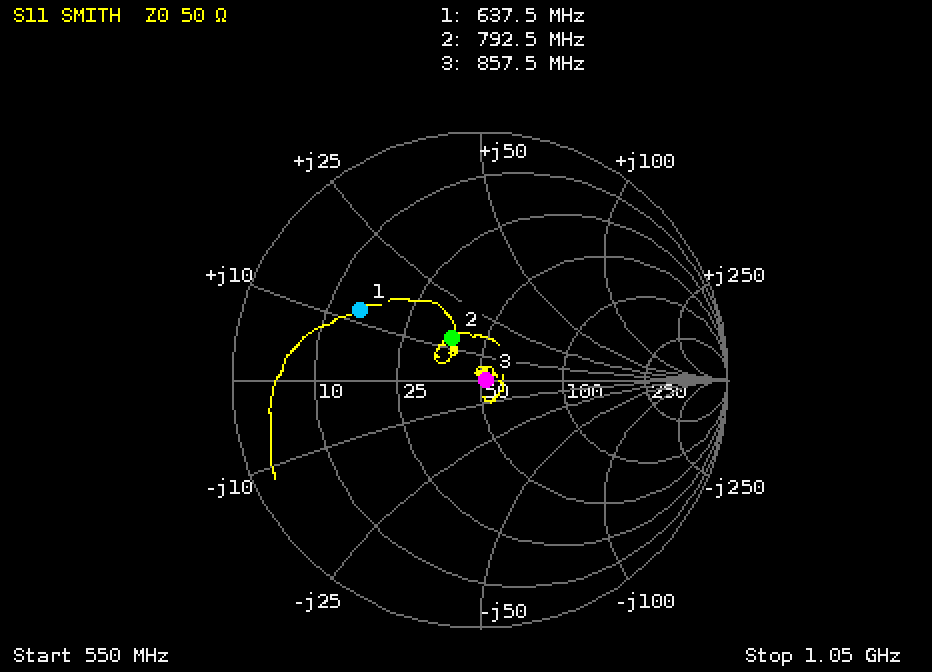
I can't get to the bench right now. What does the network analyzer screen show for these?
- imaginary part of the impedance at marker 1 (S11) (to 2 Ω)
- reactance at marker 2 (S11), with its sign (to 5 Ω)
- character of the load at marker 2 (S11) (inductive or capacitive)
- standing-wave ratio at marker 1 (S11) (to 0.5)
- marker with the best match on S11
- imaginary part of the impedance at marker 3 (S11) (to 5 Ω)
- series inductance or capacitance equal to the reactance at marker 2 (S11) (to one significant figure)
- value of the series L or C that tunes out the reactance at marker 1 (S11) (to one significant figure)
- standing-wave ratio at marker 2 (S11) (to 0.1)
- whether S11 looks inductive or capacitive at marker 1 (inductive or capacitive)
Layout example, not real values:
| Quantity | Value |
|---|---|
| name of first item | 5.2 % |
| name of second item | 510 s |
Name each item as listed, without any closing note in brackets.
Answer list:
| Quantity | Value |
|---|---|
| imaginary part of the impedance at marker 1 (S11) | +12 Ω |
| reactance at marker 2 (S11), with its sign | +15 Ω |
| character of the load at marker 2 (S11) | inductive |
| standing-wave ratio at marker 1 (S11) | 3.5 |
| marker with the best match on S11 | marker 3 |
| imaginary part of the impedance at marker 3 (S11) | 0 Ω |
| series inductance or capacitance equal to the reactance at marker 2 (S11) | 3 nH |
| value of the series L or C that tunes out the reactance at marker 1 (S11) | 20 pF |
| standing-wave ratio at marker 2 (S11) | 1.5 |
| whether S11 looks inductive or capacitive at marker 1 | inductive |
